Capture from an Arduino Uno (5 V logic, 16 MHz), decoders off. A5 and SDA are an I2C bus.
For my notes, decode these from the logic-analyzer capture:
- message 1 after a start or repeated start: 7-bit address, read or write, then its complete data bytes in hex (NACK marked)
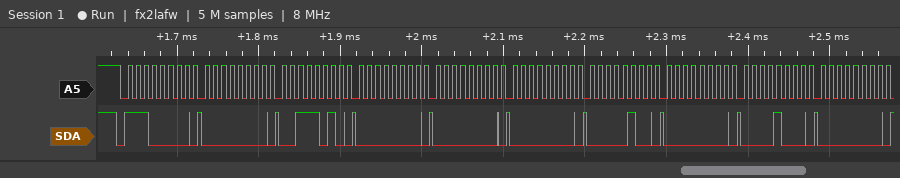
0x70 write: 00 3A 00 00 00 04 00 08 00
